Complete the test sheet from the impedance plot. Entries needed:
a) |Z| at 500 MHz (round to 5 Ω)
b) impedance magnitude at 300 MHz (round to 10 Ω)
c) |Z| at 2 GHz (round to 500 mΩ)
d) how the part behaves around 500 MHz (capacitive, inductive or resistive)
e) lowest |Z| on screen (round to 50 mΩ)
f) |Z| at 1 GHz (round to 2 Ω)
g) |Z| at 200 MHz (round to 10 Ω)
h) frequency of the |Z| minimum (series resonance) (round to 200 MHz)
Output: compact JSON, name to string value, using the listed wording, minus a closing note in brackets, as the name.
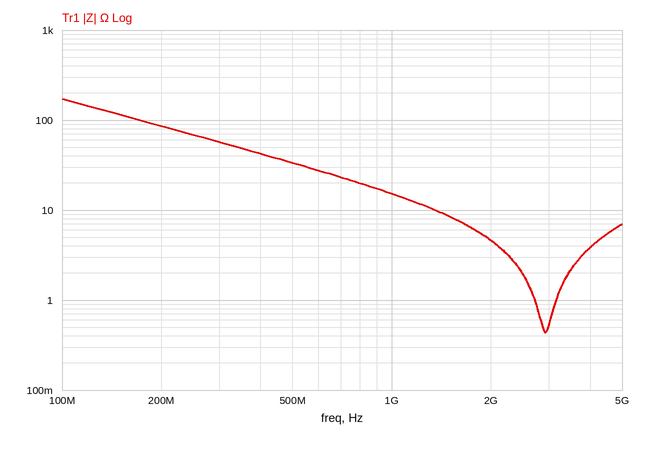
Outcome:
{"|Z| at 500 MHz": "35 Ω", "impedance magnitude at 300 MHz": "60 Ω", "|Z| at 2 GHz": "4.5 Ω", "how the part behaves around 500 MHz": "capacitive", "lowest |Z| on screen": "450 mΩ", "|Z| at 1 GHz": "16 Ω", "|Z| at 200 MHz": "90 Ω", "frequency of the |Z| minimum (series resonance)": "3.0 GHz"}
